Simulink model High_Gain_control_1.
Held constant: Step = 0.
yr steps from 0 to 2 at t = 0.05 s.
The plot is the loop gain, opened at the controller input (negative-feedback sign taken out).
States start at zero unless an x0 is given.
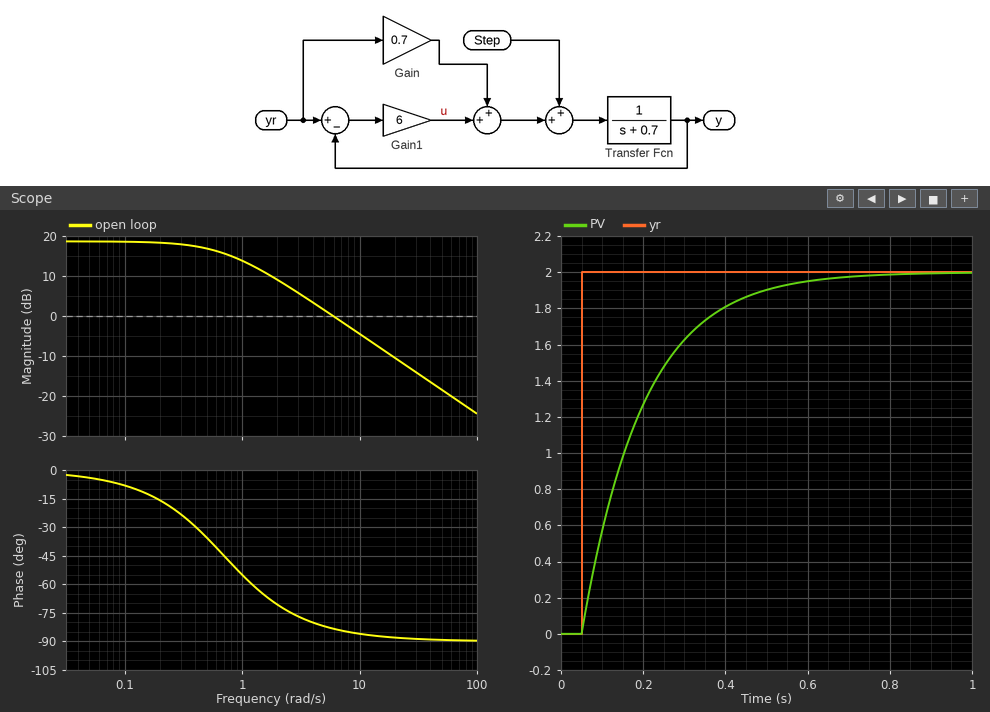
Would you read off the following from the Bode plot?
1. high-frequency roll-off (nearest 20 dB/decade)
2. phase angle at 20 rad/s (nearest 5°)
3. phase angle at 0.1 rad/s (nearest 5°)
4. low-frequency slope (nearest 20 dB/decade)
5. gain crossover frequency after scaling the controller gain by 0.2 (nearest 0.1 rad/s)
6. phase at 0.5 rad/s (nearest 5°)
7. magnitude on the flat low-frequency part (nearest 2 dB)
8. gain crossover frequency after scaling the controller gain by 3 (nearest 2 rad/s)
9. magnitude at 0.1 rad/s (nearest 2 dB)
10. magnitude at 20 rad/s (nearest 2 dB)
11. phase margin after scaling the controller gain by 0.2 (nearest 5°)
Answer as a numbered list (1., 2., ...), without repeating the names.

1. -20 dB/decade
2. -90°
3. -10°
4. 0 dB/decade
5. 1.0 rad/s
6. -35°
7. 18 dB
8. 18 rad/s
9. 18 dB
10. -10 dB
11. 125°
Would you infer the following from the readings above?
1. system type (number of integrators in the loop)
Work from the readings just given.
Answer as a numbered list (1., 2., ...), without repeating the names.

1. 0
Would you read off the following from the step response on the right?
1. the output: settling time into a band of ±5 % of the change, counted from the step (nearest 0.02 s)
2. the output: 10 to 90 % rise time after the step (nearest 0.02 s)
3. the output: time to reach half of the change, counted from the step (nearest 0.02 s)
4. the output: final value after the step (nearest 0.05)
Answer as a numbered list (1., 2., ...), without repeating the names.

1. 0.44 s
2. 0.32 s
3. 0.10 s
4. 2.00
